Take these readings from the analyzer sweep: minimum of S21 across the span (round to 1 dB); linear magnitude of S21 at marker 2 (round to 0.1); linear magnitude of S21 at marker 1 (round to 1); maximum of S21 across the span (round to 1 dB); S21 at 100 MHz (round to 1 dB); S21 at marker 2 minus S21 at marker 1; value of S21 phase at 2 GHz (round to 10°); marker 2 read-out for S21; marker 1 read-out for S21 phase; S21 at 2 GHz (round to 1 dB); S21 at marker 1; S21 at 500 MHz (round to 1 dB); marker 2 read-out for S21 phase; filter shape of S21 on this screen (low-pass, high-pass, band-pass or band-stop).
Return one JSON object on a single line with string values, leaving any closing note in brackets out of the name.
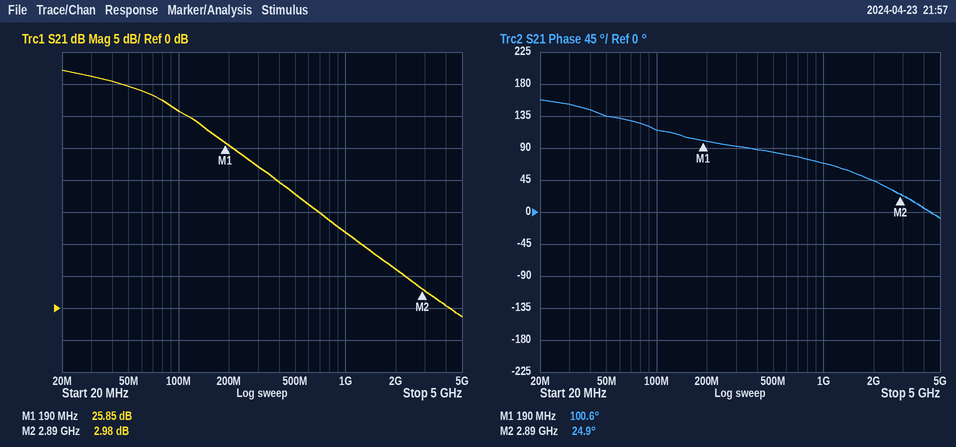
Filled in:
{"minimum of S21 across the span": "-1 dB", "linear magnitude of S21 at marker 2": "1.4", "linear magnitude of S21 at marker 1": "20", "maximum of S21 across the span": "37 dB", "S21 at 100 MHz": "31 dB", "S21 at marker 2 minus S21 at marker 1": "-22.87 dB", "value of S21 phase at 2 GHz": "40°", "marker 2 read-out for S21": "2.98 dB", "marker 1 read-out for S21 phase": "100.6°", "S21 at 2 GHz": "6 dB", "S21 at marker 1": "25.85 dB", "S21 at 500 MHz": "18 dB", "marker 2 read-out for S21 phase": "24.9°", "filter shape of S21 on this screen": "low-pass"}
